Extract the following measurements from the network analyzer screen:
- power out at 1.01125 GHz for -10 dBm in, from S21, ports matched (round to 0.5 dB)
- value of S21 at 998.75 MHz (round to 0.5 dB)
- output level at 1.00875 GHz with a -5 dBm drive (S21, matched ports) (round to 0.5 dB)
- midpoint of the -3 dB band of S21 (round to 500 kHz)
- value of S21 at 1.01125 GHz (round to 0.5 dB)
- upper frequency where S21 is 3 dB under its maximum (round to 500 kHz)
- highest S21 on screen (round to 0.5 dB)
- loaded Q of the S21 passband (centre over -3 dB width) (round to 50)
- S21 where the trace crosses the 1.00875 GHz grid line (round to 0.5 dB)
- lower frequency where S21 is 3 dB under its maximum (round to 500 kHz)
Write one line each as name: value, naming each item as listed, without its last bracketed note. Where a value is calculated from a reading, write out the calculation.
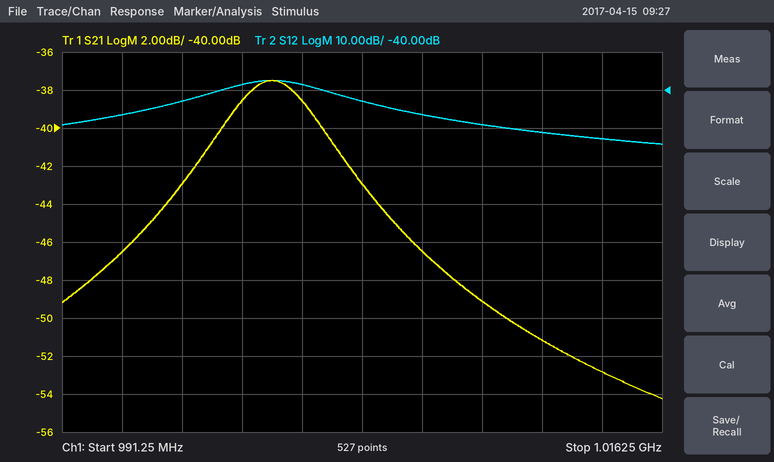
power out at 1.01125 GHz for -10 dBm in, from S21, ports matched: -10 dBm + (-51.0 dB) = -61.0 dBm
value of S21 at 998.75 MHz: -38.5 dB
output level at 1.00875 GHz with a -5 dBm drive (S21, matched ports): -5 dBm + (-49.0 dB) = -54.0 dBm
midpoint of the -3 dB band of S21: 1.0000 GHz
value of S21 at 1.01125 GHz: -51.0 dB
upper frequency where S21 is 3 dB under its maximum: 1.0025 GHz
highest S21 on screen: -37.5 dB
loaded Q of the S21 passband (centre over -3 dB width): 1 GHz / 5 MHz ≈ 200
S21 where the trace crosses the 1.00875 GHz grid line: -49.0 dB
lower frequency where S21 is 3 dB under its maximum: 997.5 MHz
